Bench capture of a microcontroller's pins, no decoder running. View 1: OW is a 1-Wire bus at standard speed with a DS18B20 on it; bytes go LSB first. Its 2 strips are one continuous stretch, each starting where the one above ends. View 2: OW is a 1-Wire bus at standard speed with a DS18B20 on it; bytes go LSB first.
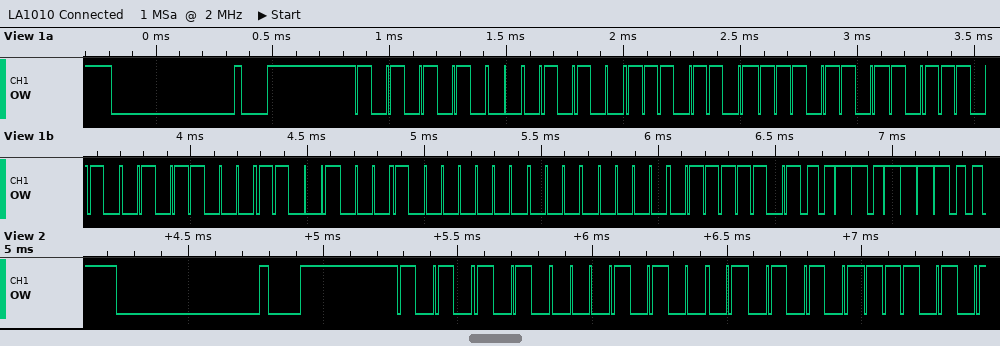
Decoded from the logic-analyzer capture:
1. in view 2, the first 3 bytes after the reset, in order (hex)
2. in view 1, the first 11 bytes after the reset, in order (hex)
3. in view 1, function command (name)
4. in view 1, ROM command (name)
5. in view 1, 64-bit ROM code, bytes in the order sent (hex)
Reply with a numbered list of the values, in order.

1. 55 28 AA
2. 55 28 B7 B7 5D 1A 13 01 00 BE EC
3. Read Scratchpad
4. Match ROM
5. 28 B7 B7 5D 1A 13 01 00
